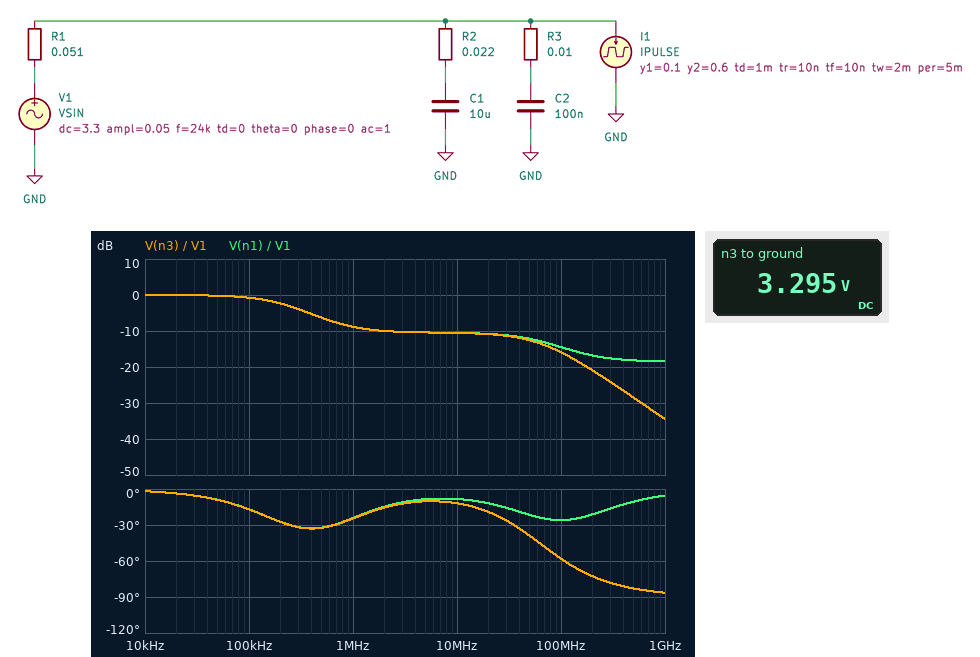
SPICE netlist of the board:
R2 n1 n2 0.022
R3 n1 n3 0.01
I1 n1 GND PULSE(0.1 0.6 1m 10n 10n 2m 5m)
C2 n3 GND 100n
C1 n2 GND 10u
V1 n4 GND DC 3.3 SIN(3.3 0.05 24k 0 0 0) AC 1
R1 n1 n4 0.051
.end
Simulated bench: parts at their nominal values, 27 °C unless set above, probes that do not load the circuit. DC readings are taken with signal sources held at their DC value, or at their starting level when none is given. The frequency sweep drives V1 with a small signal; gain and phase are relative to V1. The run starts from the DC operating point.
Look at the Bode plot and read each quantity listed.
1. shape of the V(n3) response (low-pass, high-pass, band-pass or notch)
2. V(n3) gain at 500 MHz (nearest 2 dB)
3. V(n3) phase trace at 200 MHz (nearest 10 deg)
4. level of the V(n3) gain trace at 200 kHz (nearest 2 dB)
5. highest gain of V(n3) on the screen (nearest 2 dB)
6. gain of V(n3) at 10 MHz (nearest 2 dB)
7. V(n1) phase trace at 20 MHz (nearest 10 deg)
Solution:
low-pass
-28 dB
-70 deg
-2 dB
0 dB
-10 dB
-10 deg
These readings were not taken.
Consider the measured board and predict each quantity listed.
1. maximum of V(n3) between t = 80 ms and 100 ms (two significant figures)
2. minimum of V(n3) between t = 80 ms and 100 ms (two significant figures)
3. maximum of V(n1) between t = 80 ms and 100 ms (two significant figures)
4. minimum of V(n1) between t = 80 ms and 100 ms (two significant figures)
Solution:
3.3 V
3.2 V
3.3 V
3.2 V
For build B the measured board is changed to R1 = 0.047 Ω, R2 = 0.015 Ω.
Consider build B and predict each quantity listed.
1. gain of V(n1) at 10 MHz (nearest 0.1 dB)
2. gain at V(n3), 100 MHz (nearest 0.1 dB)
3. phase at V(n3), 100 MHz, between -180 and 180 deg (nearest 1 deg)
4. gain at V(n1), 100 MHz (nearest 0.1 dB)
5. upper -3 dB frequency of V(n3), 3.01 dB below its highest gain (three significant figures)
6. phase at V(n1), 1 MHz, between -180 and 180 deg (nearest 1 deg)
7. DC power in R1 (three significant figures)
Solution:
-12.4 dB
-16.8 dB
-54 deg
-15.4 dB
271 kHz
-33 deg
470 µW
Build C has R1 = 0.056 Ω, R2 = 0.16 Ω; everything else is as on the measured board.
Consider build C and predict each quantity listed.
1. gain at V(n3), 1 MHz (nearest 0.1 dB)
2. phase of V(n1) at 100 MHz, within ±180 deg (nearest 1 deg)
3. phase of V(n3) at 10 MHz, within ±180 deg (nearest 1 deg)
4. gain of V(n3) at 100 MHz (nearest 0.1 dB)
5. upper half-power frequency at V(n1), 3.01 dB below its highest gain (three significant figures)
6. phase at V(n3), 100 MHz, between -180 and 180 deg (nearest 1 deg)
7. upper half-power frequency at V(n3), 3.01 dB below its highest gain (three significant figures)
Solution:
-2.6 dB
-41 deg
-18 deg
-13.2 dB
9.79 MHz
-73 deg
9.58 MHz
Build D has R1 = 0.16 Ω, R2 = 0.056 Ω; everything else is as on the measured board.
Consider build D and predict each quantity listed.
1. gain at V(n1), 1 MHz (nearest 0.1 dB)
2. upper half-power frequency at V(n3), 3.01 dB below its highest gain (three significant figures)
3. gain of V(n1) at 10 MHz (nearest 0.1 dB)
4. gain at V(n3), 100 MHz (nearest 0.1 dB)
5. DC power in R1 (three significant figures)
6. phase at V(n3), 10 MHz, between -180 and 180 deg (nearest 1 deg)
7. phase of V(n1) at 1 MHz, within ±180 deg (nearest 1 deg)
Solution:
-11.5 dB
78.7 kHz
-12.2 dB
-22.3 dB
1.60 mW
-19 deg
-13 deg
